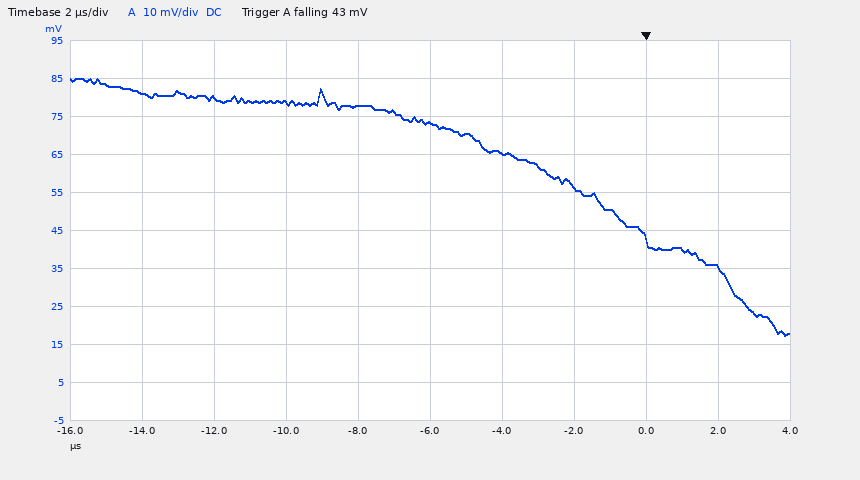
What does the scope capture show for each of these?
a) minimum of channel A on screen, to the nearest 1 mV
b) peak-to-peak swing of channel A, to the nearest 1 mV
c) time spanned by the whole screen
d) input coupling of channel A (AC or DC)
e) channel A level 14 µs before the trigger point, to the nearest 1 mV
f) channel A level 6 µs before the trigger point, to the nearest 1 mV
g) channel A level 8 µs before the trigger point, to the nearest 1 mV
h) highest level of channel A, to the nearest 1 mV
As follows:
17 mV
68 mV
20 µs
DC
81 mV
73 mV
78 mV
85 mV
